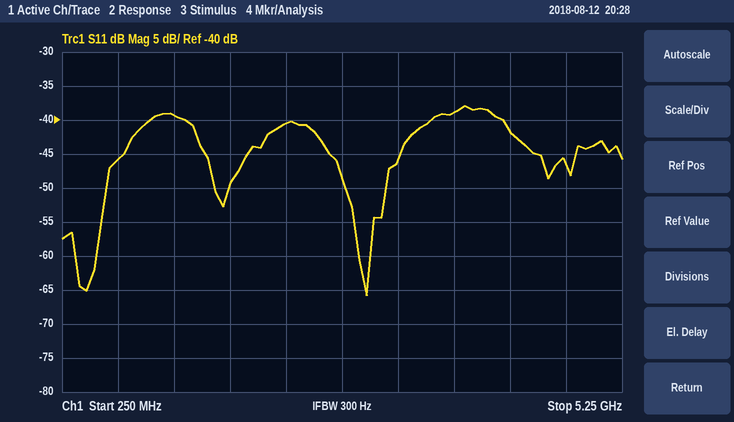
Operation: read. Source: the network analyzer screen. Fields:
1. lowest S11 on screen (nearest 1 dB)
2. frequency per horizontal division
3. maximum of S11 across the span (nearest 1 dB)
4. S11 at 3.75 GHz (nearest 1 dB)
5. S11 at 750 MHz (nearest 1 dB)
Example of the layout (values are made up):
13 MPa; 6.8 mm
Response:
-66 dB; 500 MHz; -38 dB; -39 dB; -46 dB
